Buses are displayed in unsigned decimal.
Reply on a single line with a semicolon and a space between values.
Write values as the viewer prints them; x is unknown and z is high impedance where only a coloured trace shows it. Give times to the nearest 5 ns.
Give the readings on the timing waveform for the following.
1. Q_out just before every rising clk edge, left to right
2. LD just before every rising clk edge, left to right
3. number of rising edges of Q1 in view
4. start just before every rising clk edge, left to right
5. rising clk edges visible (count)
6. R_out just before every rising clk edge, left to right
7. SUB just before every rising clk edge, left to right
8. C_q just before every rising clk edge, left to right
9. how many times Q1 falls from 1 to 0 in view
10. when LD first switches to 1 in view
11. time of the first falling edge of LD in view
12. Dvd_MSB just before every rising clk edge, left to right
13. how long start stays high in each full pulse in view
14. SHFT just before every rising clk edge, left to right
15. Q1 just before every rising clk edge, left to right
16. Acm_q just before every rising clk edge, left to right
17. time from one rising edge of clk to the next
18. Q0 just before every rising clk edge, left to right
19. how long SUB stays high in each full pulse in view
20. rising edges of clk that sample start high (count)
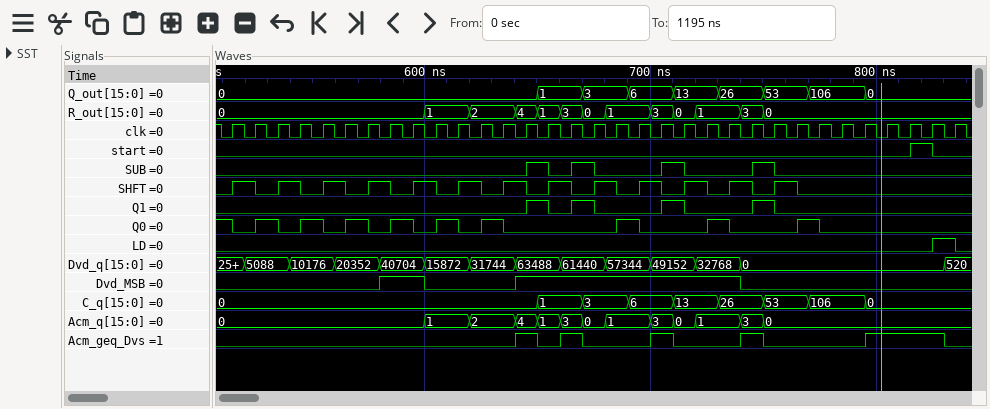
0, 0, 0, 0, 0, 0, 0, 0, 0, 0, 0, 0, 0, 0, 1, 1, 3, 3, 6, 6, 13, 13, 26, 26, 53, 53, 106, 106, 106, 0, 0, 0, 0; 0 0 0 0 0 0 0 0 0 0 0 0 0 0 0 0 0 0 0 0 0 0 0 0 0 0 0 0 0 0 0 0 1; 4; 0 0 0 0 0 0 0 0 0 0 0 0 0 0 0 0 0 0 0 0 0 0 0 0 0 0 0 0 0 0 0 1 0; 33; 0, 0, 0, 0, 0, 0, 0, 0, 0, 1, 1, 2, 2, 4, 1, 3, 0, 1, 1, 3, 0, 1, 1, 3, 0, 0, 0, 0, 0, 0, 0, 0, 0; 0 0 0 0 0 0 0 0 0 0 0 0 0 0 1 0 1 0 0 0 1 0 0 0 1 0 0 0 0 0 0 0 0; 0, 0, 0, 0, 0, 0, 0, 0, 0, 0, 0, 0, 0, 0, 1, 1, 3, 3, 6, 6, 13, 13, 26, 26, 53, 53, 106, 106, 106, 0, 0, 0, 0; 4; 825 ns; 835 ns; 0 0 0 0 0 0 0 1 1 0 0 0 0 1 1 1 1 1 1 1 1 1 1 0 0 0 0 0 0 0 0 0 0; 10 ns; 0 1 0 1 0 1 0 1 0 1 0 1 0 1 0 1 0 1 0 1 0 1 0 1 0 1 0 0 0 0 0 0 0; 0 0 0 0 0 0 0 0 0 0 0 0 0 0 1 0 1 0 0 0 1 0 0 0 1 0 0 0 0 0 0 0 0; 0, 0, 0, 0, 0, 0, 0, 0, 0, 1, 1, 2, 2, 4, 1, 3, 0, 1, 1, 3, 0, 1, 1, 3, 0, 0, 0, 0, 0, 0, 0, 0, 0; 10 ns; 1 0 1 0 1 0 1 0 1 0 1 0 1 0 0 0 0 0 1 0 0 0 1 0 0 0 1 0 0 0 0 0 0; 10 ns, 10 ns, 10 ns, 10 ns; 1
